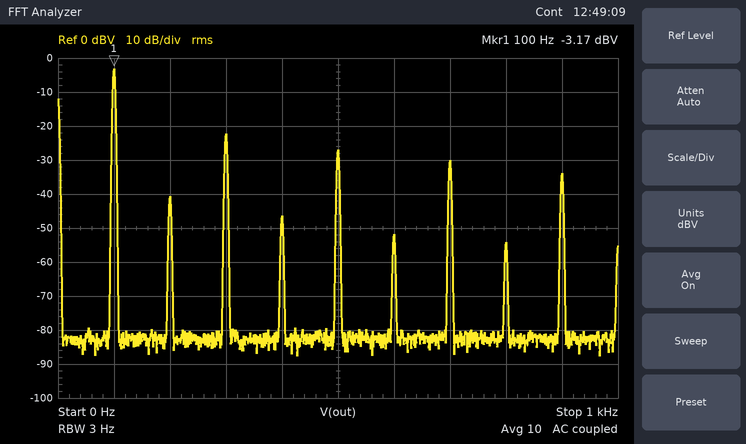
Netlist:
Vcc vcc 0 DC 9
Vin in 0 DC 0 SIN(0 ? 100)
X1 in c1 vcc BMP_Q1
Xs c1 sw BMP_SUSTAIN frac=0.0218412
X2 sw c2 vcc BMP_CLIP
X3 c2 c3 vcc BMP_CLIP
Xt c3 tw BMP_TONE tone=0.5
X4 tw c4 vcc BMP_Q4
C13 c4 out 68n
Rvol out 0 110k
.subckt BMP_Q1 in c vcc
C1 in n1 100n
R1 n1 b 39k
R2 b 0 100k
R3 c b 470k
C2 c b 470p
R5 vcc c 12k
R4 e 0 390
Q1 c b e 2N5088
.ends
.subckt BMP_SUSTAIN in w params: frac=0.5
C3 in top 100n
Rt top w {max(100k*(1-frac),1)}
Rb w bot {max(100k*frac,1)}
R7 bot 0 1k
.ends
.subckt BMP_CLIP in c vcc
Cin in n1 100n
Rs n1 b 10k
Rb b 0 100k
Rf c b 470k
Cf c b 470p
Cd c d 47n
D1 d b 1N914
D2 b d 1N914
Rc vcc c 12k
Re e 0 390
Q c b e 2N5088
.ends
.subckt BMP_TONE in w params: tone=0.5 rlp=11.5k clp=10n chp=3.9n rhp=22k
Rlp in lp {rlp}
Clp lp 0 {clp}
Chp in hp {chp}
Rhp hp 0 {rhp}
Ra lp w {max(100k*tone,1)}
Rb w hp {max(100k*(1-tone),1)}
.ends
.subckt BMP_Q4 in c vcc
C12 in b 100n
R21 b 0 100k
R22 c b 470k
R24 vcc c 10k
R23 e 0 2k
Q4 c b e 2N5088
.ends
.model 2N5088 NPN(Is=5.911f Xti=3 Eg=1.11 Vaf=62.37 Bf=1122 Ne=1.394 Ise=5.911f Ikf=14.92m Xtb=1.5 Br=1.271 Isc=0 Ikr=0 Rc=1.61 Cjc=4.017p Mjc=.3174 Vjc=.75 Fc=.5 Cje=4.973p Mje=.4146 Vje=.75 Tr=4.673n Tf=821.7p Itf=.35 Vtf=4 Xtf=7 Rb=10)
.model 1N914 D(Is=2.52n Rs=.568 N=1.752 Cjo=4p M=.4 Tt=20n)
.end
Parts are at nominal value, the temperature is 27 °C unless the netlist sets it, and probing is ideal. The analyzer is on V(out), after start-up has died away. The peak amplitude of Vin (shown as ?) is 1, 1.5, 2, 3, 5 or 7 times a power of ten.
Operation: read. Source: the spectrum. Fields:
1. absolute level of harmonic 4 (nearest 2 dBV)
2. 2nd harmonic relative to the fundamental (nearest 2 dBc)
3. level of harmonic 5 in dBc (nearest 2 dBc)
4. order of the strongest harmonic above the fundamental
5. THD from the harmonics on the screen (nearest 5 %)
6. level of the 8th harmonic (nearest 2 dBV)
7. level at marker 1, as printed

-46 dBV
-38 dBc
-24 dBc
3
15 %
-54 dBV
-3.17 dBV
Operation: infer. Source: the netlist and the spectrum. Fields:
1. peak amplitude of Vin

500 mV
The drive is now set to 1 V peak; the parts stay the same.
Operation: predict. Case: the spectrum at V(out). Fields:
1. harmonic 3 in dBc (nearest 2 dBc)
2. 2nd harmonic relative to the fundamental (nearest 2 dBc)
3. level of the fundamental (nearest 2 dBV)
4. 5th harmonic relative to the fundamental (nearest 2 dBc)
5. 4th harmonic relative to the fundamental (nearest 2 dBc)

-22 dBc
-24 dBc
-2 dBV
-26 dBc
-28 dBc
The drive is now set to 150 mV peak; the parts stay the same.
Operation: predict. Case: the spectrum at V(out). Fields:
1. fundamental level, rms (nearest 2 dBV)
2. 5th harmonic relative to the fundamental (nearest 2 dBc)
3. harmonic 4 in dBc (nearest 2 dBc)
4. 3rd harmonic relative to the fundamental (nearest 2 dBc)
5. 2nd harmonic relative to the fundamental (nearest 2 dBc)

-6 dBV
-22 dBc
-56 dBc
-16 dBc
-46 dBc
